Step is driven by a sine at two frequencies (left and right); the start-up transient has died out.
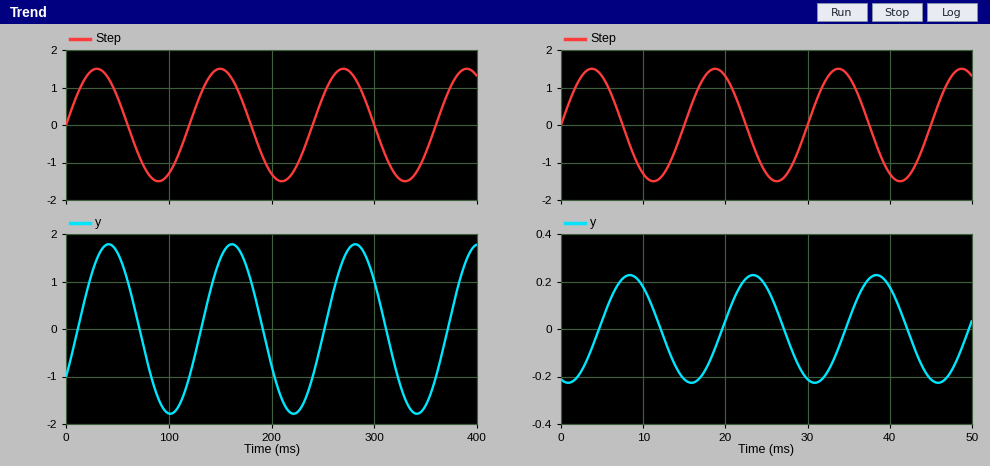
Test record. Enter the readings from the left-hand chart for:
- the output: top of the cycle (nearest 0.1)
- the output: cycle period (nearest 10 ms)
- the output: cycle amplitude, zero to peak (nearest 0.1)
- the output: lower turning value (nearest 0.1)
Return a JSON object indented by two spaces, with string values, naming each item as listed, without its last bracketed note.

{
  "the output: top of the cycle": "1.8",
  "the output: cycle period": "120 ms",
  "the output: cycle amplitude, zero to peak": "1.8",
  "the output: lower turning value": "-1.8"
}
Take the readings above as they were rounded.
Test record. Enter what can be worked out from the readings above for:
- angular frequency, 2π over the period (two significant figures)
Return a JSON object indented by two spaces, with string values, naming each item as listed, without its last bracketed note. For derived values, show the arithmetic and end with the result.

{
  "angular frequency, 2π over the period": "2π / 120 = 0.052 rad/ms"
}
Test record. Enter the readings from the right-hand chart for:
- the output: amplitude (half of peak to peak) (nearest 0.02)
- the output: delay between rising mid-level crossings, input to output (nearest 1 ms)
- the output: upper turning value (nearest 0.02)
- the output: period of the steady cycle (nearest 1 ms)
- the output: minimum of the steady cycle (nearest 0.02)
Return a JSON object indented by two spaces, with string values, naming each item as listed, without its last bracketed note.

{
  "the output: amplitude (half of peak to peak)": "0.22",
  "the output: delay between rising mid-level crossings, input to output": "5 ms",
  "the output: upper turning value": "0.22",
  "the output: period of the steady cycle": "15 ms",
  "the output: minimum of the steady cycle": "-0.22"
}
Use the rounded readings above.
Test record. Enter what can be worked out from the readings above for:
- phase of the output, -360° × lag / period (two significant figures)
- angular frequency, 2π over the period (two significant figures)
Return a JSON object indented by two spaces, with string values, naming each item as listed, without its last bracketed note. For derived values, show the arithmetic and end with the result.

{
  "phase of the output, -360° × lag / period": "-360 × 5 / 15 = -120°",
  "angular frequency, 2π over the period": "2π / 15 = 0.42 rad/ms"
}
